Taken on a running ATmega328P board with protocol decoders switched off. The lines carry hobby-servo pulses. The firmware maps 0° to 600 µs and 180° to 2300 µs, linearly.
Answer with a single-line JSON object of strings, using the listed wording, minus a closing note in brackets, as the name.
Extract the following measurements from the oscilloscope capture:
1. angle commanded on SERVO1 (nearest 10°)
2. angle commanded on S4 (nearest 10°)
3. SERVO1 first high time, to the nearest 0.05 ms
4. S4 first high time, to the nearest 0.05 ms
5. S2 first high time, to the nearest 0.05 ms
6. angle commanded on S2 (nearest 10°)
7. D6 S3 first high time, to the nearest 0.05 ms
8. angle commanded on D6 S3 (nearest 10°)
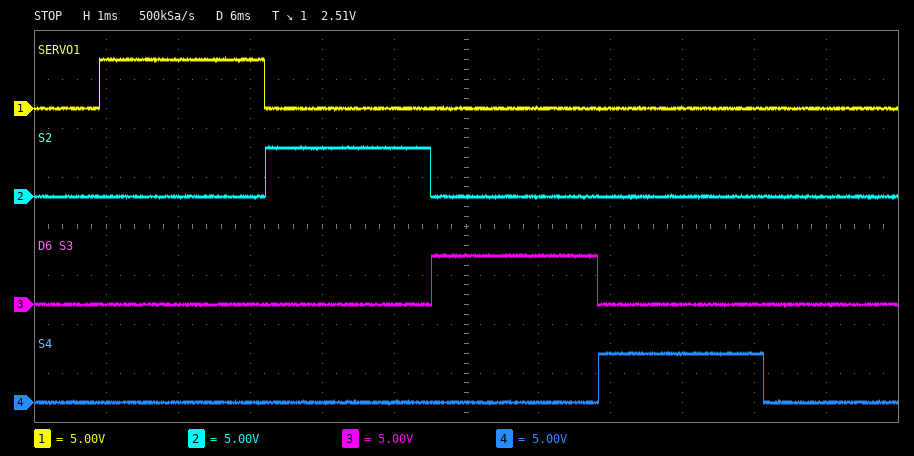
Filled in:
{"angle commanded on SERVO1": "180°", "angle commanded on S4": "180°", "SERVO1 first high time, to the nearest 0.05 ms": "2.30 ms", "S4 first high time, to the nearest 0.05 ms": "2.30 ms", "S2 first high time, to the nearest 0.05 ms": "2.30 ms", "angle commanded on S2": "180°", "D6 S3 first high time, to the nearest 0.05 ms": "2.30 ms", "angle commanded on D6 S3": "180°"}
